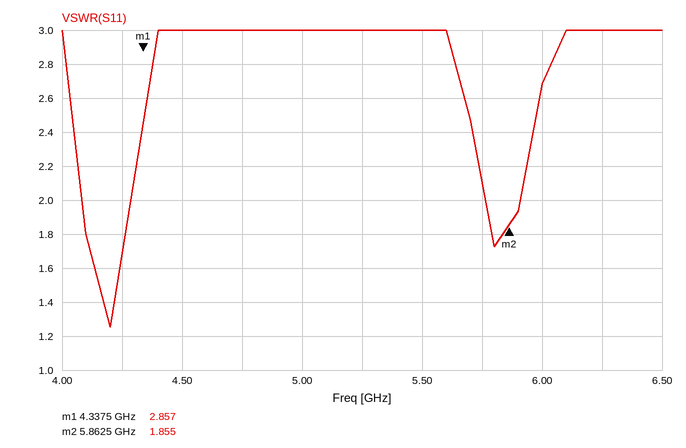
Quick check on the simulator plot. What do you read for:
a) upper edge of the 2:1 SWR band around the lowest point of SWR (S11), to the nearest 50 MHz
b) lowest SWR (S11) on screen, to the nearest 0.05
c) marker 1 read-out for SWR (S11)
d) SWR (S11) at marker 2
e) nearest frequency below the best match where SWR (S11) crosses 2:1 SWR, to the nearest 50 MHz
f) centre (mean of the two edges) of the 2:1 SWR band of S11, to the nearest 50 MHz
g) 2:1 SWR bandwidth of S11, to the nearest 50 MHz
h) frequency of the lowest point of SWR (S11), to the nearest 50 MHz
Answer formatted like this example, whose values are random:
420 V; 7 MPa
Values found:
4.30 GHz; 1.25; 2.857; 1.855; 4.10 GHz; 4.20 GHz; 200 MHz; 4.20 GHz
